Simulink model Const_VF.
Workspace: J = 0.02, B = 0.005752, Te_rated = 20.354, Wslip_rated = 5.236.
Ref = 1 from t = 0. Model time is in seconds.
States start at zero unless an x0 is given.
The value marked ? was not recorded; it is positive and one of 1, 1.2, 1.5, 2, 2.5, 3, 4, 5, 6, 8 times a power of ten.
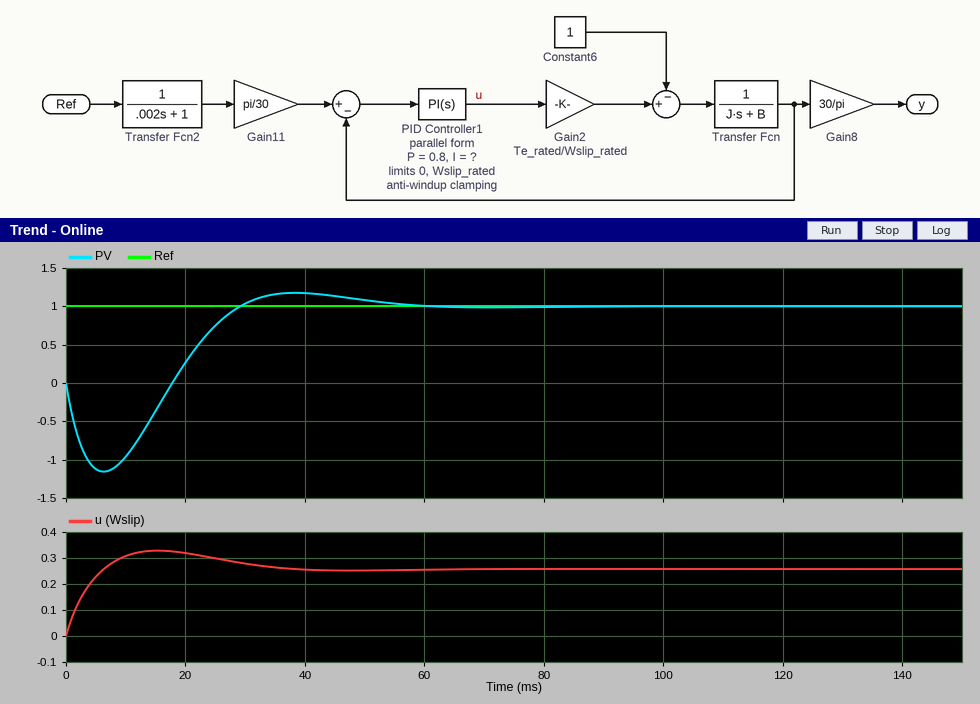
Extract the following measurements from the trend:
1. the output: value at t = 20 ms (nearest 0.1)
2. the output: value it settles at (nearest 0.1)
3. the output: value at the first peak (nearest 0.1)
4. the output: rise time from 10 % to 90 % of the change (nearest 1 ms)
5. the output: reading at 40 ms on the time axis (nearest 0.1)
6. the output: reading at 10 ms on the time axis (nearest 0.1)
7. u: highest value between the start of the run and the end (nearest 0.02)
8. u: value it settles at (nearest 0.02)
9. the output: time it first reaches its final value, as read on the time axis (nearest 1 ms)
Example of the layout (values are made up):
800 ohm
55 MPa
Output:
0.3
1.0
1.2
9 ms
1.2
-1.0
0.32
0.26
29 ms
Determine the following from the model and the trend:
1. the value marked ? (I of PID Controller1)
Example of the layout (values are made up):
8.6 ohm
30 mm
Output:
80
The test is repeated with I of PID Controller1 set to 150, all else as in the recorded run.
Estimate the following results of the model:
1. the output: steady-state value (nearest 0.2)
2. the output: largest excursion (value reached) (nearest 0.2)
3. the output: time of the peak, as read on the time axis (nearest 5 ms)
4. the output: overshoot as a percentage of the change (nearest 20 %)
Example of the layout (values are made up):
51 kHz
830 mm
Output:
1.0
1.4
25 ms
40 %
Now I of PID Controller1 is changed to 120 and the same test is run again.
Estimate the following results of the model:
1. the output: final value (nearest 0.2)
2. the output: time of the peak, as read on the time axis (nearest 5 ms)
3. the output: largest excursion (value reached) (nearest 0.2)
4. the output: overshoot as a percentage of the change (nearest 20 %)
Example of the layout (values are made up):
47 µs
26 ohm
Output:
1.0
30 ms
1.4
40 %
